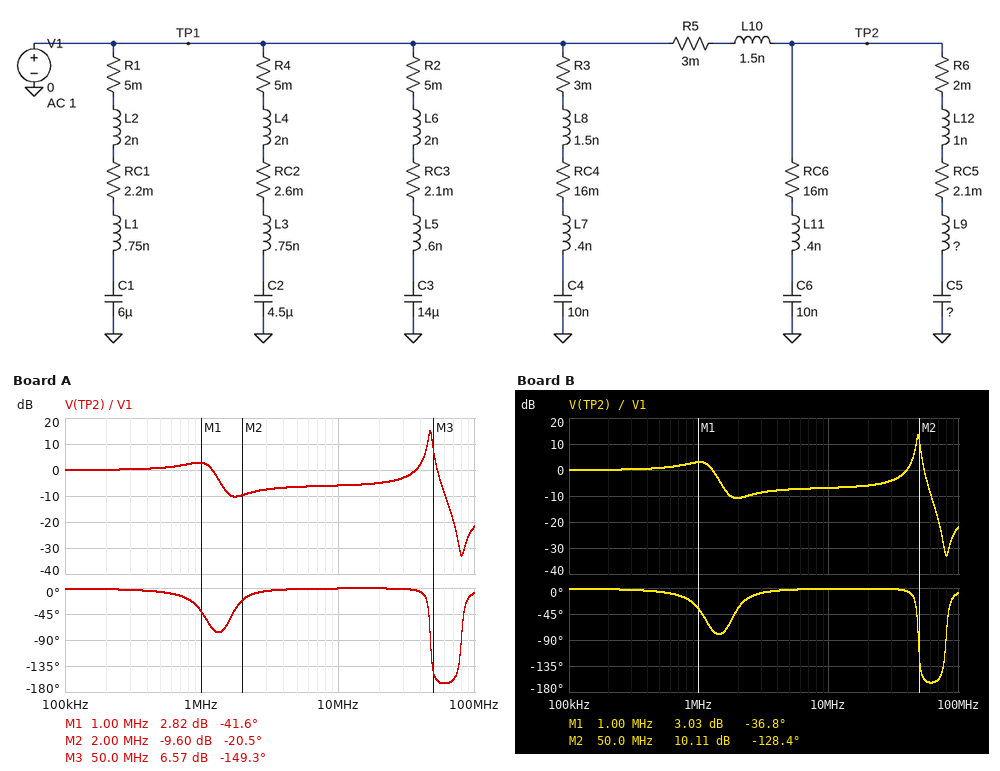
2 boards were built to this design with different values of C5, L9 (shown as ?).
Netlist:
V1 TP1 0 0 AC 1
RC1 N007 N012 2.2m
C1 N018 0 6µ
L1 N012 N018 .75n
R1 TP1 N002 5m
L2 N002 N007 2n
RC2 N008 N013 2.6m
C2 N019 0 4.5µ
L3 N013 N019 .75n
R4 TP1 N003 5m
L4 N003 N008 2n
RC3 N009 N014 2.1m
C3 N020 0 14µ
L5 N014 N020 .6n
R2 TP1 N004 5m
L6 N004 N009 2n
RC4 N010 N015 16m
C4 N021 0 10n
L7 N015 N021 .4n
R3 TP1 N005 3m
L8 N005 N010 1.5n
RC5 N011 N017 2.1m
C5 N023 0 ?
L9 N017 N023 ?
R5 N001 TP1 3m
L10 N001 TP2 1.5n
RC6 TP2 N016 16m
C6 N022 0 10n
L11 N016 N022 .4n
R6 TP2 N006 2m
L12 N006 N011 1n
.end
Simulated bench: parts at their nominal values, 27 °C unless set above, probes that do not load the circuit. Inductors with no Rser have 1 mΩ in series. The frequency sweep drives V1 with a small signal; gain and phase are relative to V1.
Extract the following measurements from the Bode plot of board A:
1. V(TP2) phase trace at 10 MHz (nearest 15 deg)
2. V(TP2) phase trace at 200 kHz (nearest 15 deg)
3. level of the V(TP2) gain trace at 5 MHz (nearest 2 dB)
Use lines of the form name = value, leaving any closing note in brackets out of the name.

V(TP2) phase trace at 10 MHz = 0 deg
V(TP2) phase trace at 200 kHz = 0 deg
level of the V(TP2) gain trace at 5 MHz = -6 dB
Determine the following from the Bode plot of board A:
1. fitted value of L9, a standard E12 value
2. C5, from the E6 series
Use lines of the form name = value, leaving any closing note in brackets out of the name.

fitted value of L9, a standard E12 value = 470 pH
C5, from the E6 series = 6.8 µF
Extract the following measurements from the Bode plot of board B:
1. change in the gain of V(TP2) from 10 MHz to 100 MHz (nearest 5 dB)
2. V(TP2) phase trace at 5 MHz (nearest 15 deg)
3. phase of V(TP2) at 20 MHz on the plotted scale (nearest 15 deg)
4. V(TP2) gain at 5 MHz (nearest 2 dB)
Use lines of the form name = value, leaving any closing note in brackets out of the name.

change in the gain of V(TP2) from 10 MHz to 100 MHz = -15 dB
V(TP2) phase trace at 5 MHz = 0 deg
phase of V(TP2) at 20 MHz on the plotted scale = 0 deg
V(TP2) gain at 5 MHz = -8 dB
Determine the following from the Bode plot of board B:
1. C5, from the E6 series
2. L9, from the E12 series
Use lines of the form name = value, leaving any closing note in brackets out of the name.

C5, from the E6 series = 6.8 µF
L9, from the E12 series = 220 pH
